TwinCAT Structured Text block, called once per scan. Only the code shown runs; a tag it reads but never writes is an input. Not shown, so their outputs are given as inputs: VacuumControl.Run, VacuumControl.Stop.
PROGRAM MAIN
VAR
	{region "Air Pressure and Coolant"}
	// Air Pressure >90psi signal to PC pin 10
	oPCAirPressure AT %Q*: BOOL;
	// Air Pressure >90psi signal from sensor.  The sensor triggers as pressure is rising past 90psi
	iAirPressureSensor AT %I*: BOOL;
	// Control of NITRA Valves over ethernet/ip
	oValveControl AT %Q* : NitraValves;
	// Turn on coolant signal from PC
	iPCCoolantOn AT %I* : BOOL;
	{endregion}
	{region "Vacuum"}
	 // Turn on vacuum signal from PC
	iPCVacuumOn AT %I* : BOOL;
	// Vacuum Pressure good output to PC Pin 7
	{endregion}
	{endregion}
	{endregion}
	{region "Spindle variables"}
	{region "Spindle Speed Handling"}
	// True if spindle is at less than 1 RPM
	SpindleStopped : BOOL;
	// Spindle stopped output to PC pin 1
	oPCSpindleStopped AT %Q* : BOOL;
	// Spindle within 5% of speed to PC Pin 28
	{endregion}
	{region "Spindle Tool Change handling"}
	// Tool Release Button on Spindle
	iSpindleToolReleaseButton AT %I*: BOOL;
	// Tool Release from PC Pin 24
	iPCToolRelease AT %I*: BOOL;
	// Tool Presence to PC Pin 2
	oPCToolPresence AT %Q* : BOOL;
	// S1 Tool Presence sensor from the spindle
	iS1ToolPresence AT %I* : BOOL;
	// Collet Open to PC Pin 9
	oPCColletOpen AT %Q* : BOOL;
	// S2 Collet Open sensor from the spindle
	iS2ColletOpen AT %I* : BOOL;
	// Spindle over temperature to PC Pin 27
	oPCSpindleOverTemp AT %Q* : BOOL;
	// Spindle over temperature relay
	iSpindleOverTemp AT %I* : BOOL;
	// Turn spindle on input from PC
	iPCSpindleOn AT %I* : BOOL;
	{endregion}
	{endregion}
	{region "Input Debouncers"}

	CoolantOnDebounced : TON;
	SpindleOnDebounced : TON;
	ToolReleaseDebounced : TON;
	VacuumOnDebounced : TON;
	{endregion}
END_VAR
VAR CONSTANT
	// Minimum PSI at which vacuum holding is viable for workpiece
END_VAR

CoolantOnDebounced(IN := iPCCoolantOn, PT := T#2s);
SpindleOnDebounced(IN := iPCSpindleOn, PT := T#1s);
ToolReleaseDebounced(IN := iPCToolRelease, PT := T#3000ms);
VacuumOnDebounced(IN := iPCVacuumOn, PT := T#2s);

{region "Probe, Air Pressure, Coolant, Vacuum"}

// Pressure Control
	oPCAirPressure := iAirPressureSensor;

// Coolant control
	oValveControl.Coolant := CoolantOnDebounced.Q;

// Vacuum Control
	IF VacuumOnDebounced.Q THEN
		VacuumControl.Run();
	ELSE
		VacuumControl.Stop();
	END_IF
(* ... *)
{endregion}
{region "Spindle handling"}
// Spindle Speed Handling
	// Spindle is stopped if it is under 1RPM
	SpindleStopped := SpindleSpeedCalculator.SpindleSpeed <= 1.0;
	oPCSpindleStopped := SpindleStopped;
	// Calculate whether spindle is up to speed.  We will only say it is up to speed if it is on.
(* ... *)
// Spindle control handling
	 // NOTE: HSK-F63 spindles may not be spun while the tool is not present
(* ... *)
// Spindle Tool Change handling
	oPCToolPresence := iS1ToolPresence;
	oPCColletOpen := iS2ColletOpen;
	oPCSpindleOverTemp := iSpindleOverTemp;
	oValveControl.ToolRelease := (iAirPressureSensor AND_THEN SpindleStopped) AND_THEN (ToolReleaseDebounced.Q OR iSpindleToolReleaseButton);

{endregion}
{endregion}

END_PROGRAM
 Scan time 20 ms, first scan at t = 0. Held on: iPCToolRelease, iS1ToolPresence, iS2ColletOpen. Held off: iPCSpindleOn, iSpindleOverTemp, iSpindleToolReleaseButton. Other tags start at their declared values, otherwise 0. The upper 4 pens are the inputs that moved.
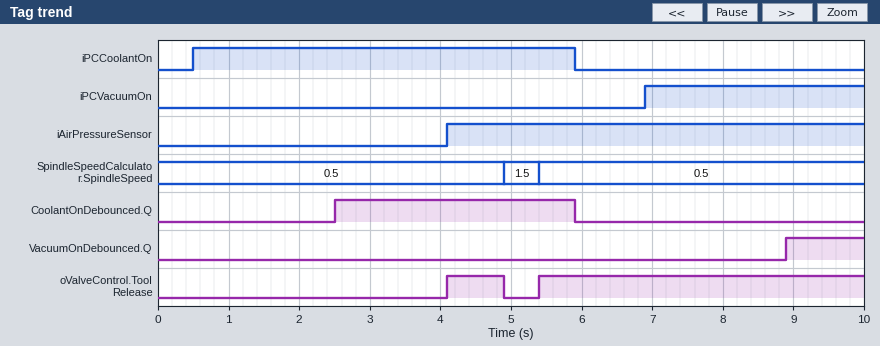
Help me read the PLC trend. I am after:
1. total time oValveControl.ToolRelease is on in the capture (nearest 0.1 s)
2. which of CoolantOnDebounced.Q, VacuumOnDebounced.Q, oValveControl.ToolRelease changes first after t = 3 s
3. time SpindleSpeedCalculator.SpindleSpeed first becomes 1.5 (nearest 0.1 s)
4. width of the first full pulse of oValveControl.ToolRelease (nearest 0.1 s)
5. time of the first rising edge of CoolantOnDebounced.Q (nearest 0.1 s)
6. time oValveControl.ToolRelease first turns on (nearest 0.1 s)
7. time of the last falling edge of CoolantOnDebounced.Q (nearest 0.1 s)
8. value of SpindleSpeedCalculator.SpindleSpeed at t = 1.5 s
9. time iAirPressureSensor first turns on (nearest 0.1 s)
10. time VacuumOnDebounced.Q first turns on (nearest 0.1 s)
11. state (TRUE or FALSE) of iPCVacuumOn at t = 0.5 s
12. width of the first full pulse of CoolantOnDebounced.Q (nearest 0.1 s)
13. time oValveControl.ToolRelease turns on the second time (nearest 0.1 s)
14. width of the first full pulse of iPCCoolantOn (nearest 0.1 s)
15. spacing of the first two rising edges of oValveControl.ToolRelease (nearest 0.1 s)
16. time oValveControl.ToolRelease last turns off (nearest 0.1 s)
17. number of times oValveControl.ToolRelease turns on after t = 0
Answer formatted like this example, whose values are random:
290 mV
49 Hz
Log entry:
5.4 s
oValveControl.ToolRelease
4.9 s
0.8 s
2.5 s
4.1 s
5.9 s
0.5
4.1 s
8.9 s
FALSE
3.4 s
5.4 s
5.4 s
1.3 s
4.9 s
2
